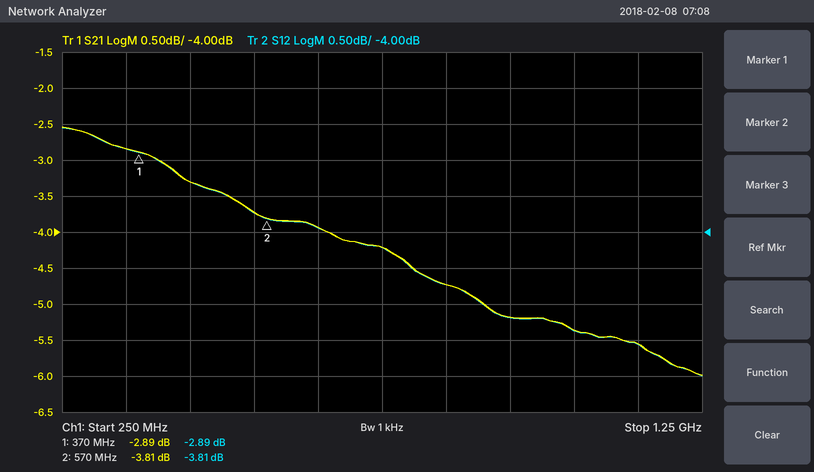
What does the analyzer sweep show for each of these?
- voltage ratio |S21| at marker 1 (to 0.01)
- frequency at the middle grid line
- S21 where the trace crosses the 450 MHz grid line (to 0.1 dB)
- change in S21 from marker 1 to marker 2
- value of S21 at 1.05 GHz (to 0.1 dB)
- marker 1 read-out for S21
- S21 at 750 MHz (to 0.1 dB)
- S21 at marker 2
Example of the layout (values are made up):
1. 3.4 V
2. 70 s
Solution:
1. 0.72
2. 750 MHz
3. -3.3 dB
4. -0.92 dB
5. -5.4 dB
6. -2.89 dB
7. -4.2 dB
8. -3.81 dB
